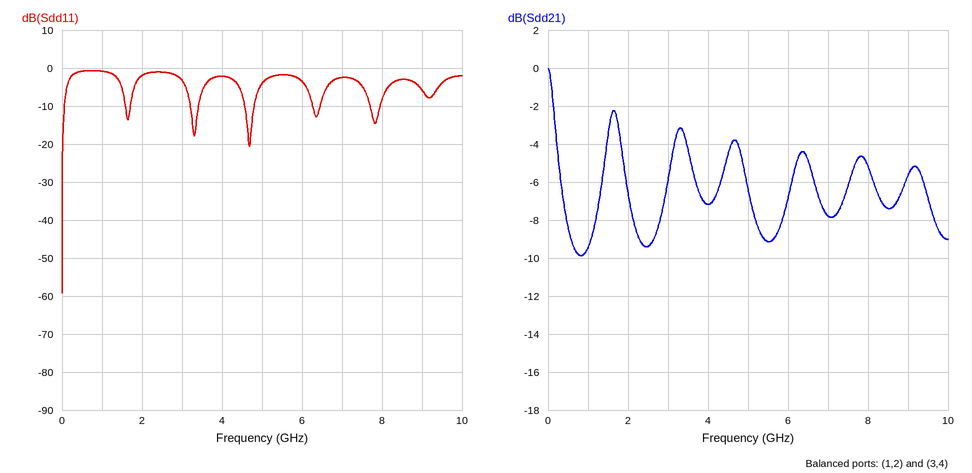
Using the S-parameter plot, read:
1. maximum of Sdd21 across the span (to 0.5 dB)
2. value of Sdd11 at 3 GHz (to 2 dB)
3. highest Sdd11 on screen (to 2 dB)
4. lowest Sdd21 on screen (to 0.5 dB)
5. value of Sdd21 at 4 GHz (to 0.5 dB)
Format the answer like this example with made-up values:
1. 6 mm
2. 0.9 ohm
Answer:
1. 0.0 dB
2. -4 dB
3. 0 dB
4. -10.0 dB
5. -7.0 dB
